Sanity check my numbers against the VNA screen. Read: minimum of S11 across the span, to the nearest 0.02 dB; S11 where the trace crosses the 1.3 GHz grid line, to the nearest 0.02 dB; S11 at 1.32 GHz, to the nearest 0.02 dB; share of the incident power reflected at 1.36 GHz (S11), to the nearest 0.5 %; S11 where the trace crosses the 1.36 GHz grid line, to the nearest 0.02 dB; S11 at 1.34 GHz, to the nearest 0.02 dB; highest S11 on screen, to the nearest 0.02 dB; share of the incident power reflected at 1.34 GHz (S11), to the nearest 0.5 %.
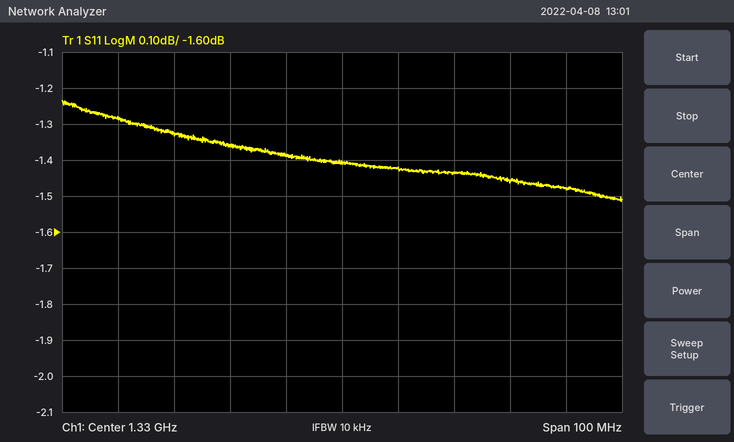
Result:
-1.52 dB
-1.32 dB
-1.38 dB
71.5 %
-1.46 dB
-1.42 dB
-1.24 dB
72.0 %
